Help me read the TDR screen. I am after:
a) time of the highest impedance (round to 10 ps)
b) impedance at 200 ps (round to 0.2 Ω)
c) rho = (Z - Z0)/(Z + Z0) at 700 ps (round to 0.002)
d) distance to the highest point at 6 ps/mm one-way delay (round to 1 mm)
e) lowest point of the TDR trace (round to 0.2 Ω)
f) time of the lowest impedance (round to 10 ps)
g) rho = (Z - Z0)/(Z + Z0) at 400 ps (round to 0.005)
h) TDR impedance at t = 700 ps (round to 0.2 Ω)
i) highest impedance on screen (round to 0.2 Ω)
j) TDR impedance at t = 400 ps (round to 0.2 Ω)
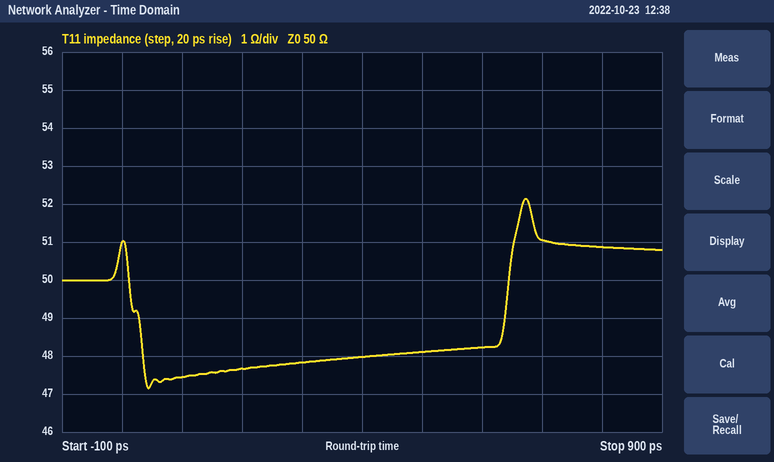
670 ps
47.6 Ω
+0.010
56 mm
47.2 Ω
40 ps
-0.020
51.0 Ω
52.2 Ω
48.0 Ω
